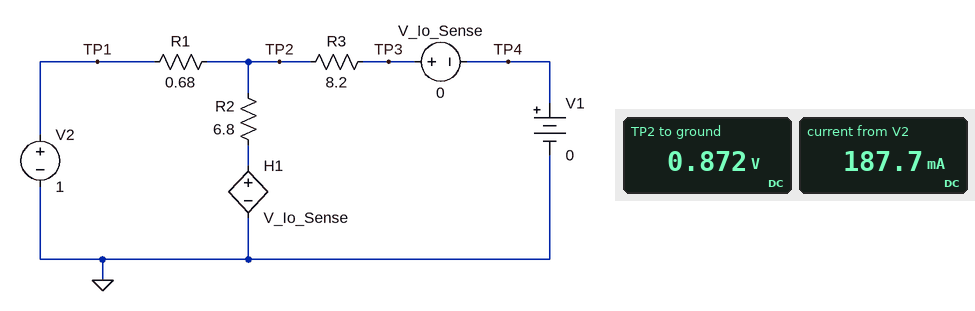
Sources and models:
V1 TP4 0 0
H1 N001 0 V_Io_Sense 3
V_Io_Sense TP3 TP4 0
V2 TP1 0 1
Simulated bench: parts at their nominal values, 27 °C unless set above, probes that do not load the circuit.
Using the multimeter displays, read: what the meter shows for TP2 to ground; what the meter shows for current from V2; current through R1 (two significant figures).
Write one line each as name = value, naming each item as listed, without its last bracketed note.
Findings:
what the meter shows for TP2 to ground = 0.872 V
what the meter shows for current from V2 = 187.7 mA
current through R1 = 190 mA
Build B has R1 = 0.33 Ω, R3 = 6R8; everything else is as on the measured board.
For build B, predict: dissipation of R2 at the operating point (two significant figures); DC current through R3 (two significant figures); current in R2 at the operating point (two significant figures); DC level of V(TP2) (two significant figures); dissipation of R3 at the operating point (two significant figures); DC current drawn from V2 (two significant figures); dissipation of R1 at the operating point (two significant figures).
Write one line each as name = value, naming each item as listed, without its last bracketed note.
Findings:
dissipation of R2 at the operating point = 40 mW
DC current through R3 = 140 mA
current in R2 at the operating point = 76 mA
DC level of V(TP2) = 930 mV
dissipation of R3 at the operating point = 130 mW
DC current drawn from V2 = 210 mA
dissipation of R1 at the operating point = 15 mW
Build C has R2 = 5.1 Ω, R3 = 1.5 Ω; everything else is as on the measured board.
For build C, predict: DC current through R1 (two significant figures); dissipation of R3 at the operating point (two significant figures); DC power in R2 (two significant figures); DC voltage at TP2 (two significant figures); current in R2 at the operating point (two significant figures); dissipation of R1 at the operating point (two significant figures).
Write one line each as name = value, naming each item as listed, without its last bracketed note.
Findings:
DC current through R1 = 360 mA
dissipation of R3 at the operating point = 380 mW
DC power in R2 = 110 mW
DC voltage at TP2 = 760 mV
current in R2 at the operating point = 150 mA
dissipation of R1 at the operating point = 86 mW
